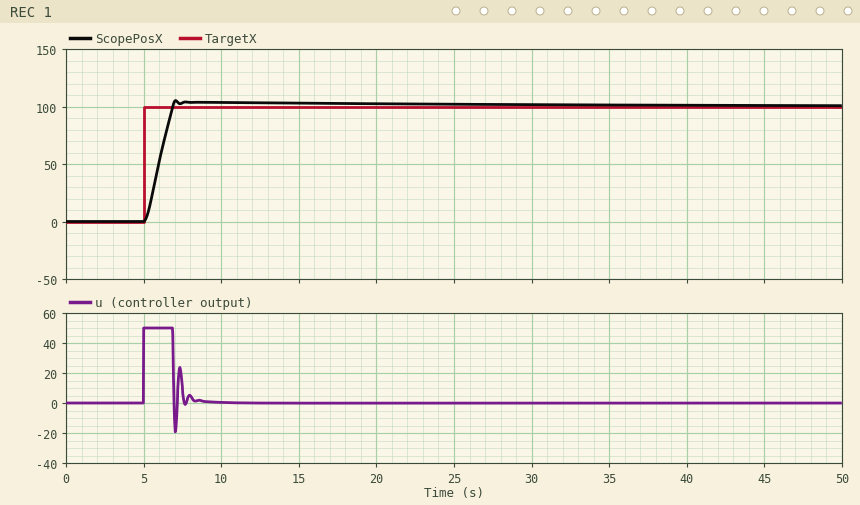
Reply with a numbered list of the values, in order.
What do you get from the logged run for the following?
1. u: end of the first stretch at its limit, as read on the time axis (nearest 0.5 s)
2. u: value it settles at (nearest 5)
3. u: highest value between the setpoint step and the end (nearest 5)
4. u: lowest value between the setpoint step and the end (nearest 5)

1. 7.0 s
2. 0
3. 50
4. -20
